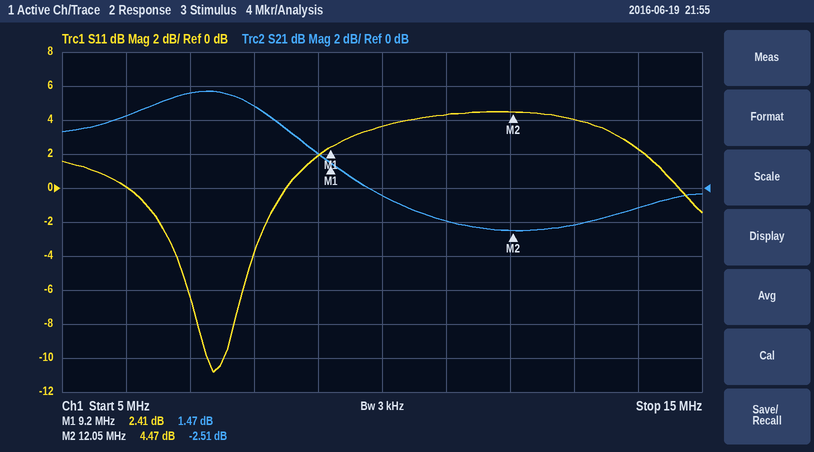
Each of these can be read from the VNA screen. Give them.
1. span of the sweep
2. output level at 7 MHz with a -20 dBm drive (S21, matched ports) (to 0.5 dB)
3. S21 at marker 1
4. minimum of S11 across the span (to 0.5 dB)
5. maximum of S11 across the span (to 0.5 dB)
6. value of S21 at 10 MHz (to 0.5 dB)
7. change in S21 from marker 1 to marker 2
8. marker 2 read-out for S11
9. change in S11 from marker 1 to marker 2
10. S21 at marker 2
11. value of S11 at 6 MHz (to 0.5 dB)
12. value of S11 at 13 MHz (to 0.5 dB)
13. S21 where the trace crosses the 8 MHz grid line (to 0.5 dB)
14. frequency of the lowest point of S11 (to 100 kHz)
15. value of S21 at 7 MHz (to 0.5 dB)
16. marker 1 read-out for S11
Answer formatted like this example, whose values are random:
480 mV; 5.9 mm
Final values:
10 MHz; -14.5 dBm; 1.47 dB; -11.0 dB; 4.5 dB; -0.5 dB; -3.98 dB; 4.47 dB; 2.06 dB; -2.51 dB; 0.0 dB; 4.0 dB; 5.0 dB; 7.4 MHz; 5.5 dB; 2.41 dB
